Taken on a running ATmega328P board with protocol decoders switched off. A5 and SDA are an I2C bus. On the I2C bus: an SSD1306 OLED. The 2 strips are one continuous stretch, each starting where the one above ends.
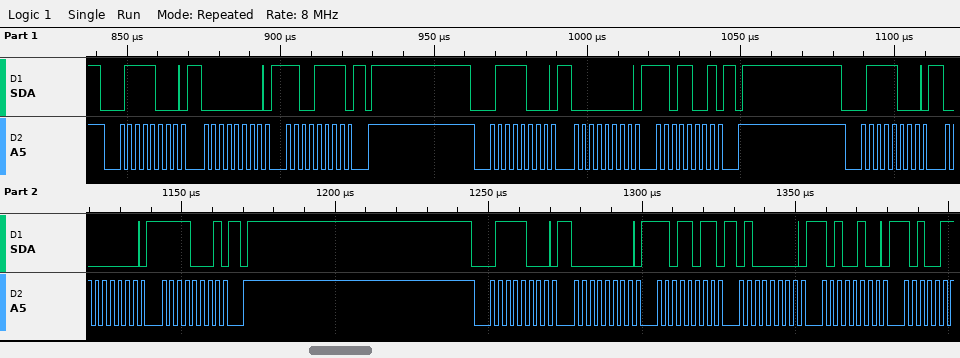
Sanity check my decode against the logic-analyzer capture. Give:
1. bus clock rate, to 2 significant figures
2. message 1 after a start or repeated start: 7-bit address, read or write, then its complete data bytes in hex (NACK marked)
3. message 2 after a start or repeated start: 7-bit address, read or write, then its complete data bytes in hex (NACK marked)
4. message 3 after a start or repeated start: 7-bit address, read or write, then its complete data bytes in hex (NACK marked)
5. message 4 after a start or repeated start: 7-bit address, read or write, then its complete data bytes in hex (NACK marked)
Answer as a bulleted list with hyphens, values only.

- 400 kHz
- 0x3C write: 00 CF
- 0x3C write: 00 D9
- 0x3C write: 00 F1
- 0x3C write: 00 DB 40 A4
